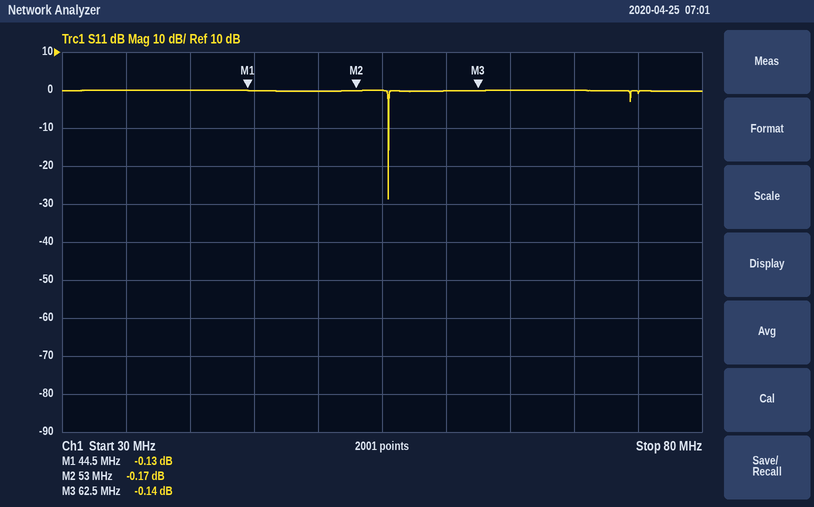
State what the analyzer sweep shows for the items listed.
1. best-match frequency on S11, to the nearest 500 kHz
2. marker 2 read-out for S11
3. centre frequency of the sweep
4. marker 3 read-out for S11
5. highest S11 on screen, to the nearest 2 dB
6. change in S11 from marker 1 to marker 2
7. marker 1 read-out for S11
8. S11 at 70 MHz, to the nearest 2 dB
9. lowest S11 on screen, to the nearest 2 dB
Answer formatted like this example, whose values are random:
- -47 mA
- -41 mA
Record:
- 55.5 MHz
- -0.17 dB
- 55 MHz
- -0.14 dB
- 0 dB
- -0.04 dB
- -0.13 dB
- 0 dB
- -28 dB
